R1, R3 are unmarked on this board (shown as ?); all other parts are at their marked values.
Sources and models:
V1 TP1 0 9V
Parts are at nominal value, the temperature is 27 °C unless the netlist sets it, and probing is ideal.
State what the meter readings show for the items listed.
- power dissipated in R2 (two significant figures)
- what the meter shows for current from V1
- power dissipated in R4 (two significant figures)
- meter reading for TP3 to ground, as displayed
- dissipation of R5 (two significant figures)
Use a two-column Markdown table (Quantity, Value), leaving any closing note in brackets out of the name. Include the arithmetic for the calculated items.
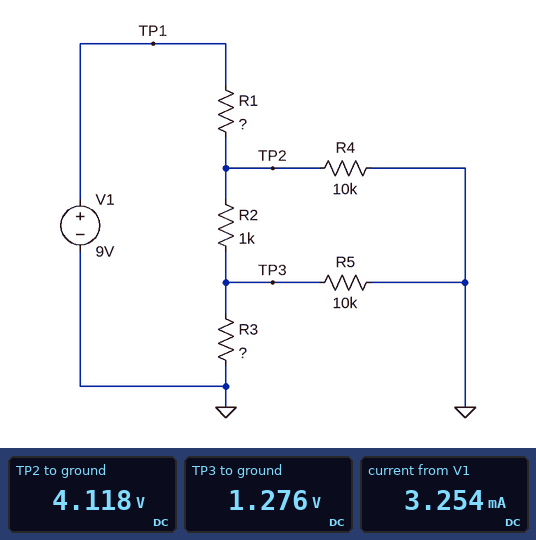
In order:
| Quantity | Value |
|---|---|
| power dissipated in R2 | (4.118 V - 1.276 V)^2 / 1 kΩ = 8.1 mW |
| what the meter shows for current from V1 | 3.254 mA |
| power dissipated in R4 | (4.118 V)^2 / 10 kΩ = 1.7 mW |
| meter reading for TP3 to ground, as displayed | 1.276 V |
| dissipation of R5 | (1.276 V)^2 / 10 kΩ = 160 µW |
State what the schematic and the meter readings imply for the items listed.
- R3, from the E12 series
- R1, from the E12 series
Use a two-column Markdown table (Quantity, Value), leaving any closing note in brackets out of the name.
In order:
| Quantity | Value |
|---|---|
| R3, from the E12 series | 470 Ω |
| R1, from the E12 series | 1.5 kΩ |
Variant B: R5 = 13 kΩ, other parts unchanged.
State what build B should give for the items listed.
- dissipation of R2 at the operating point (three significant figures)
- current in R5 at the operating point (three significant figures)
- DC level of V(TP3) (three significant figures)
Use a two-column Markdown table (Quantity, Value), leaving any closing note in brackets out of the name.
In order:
| Quantity | Value |
|---|---|
| dissipation of R2 at the operating point | 8.05 mW |
| current in R5 at the operating point | 99.0 µA |
| DC level of V(TP3) | 1.29 V |
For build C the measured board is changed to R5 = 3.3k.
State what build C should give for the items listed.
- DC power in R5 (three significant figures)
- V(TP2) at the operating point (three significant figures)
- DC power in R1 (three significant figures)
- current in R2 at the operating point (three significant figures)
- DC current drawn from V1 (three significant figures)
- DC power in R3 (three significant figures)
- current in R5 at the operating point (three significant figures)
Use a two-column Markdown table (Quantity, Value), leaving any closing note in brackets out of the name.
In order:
| Quantity | Value |
|---|---|
| DC power in R5 | 426 µW |
| V(TP2) at the operating point | 4.07 V |
| DC power in R1 | 16.2 mW |
| current in R2 at the operating point | 2.88 mA |
| DC current drawn from V1 | 3.29 mA |
| DC power in R3 | 2.99 mW |
| current in R5 at the operating point | 359 µA |
